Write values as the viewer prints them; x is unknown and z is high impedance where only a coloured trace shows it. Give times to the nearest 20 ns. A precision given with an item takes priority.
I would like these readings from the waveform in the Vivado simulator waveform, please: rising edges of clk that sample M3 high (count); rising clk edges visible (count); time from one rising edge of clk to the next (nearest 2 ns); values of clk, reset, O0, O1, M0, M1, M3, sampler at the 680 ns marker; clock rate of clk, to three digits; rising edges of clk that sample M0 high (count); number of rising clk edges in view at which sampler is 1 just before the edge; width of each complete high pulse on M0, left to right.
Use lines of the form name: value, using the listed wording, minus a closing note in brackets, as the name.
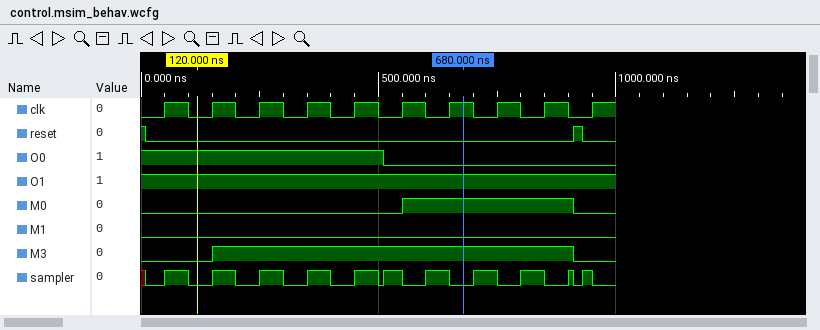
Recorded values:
rising edges of clk that sample M3 high: 7
rising clk edges visible: 10
time from one rising edge of clk to the next: 100 ns
values of clk, reset, O0, O1, M0, M1, M3, sampler at the 680 ns marker: clk=1, reset=0, O0=0, O1=1, M0=1, M1=0, M3=1, sampler=0
clock rate of clk, to three digits: 10.0 MHz
rising edges of clk that sample M0 high: 3
number of rising clk edges in view at which sampler is 1 just before the edge: 5
width of each complete high pulse on M0, left to right: 360 ns
